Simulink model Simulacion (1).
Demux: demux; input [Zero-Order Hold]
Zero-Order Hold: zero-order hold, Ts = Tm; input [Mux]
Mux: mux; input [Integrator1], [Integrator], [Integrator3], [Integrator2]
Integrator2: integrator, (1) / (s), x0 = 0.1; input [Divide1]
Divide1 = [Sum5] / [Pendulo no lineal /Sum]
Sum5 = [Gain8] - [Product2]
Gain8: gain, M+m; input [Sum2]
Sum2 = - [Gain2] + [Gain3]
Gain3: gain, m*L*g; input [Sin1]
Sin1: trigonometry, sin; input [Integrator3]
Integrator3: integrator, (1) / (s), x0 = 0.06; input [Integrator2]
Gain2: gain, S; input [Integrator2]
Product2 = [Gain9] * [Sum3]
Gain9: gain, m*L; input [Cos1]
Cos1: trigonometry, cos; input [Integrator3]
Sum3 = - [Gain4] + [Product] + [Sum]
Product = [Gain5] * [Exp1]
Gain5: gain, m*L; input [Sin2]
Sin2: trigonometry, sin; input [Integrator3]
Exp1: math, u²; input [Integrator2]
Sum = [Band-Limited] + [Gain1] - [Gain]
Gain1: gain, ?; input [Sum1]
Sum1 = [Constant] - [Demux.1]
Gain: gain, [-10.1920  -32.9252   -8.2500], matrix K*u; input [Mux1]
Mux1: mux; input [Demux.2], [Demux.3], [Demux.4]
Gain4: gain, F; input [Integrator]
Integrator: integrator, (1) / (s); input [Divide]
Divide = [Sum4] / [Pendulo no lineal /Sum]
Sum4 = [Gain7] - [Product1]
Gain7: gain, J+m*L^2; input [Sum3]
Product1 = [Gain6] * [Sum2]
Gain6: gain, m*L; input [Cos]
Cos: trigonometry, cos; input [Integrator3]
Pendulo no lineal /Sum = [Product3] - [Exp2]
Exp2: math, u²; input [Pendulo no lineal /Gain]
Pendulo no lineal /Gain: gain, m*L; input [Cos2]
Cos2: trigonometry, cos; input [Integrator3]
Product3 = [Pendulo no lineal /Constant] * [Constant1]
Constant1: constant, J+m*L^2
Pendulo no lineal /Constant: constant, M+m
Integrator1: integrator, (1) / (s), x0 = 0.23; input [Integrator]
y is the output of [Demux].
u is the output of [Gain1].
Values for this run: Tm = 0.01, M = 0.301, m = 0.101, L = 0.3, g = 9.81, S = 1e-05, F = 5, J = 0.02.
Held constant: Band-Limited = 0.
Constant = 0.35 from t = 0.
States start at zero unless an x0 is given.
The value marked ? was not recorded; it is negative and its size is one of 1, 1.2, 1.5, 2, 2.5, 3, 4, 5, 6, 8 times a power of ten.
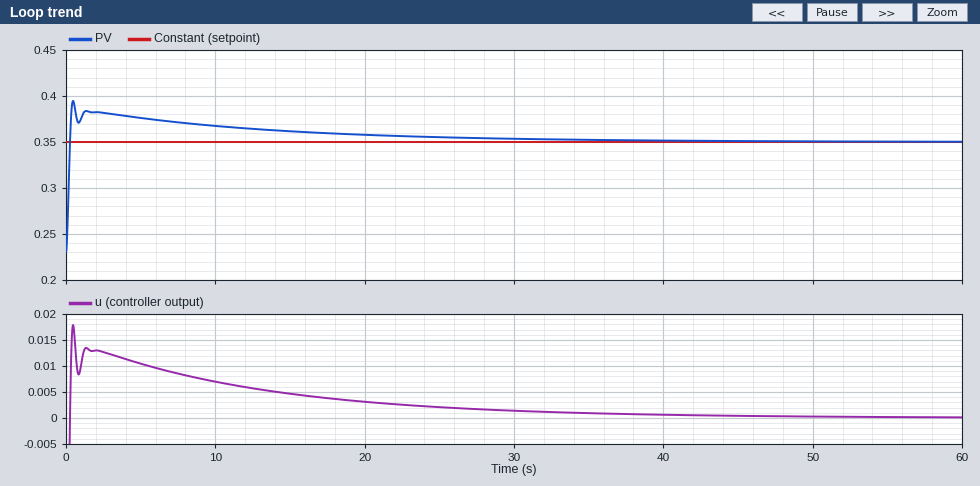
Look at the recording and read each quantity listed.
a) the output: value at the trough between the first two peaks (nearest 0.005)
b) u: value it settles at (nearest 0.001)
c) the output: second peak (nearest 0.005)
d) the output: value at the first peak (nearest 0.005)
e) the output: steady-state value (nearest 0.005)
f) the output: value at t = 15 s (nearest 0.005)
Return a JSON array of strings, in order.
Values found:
["0.370", "0.000", "0.385", "0.395", "0.350", "0.360"]
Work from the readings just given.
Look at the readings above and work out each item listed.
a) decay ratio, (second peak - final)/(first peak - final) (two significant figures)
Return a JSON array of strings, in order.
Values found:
["0.78"]
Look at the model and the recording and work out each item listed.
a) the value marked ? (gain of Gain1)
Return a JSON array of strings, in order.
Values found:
["-0.4"]
